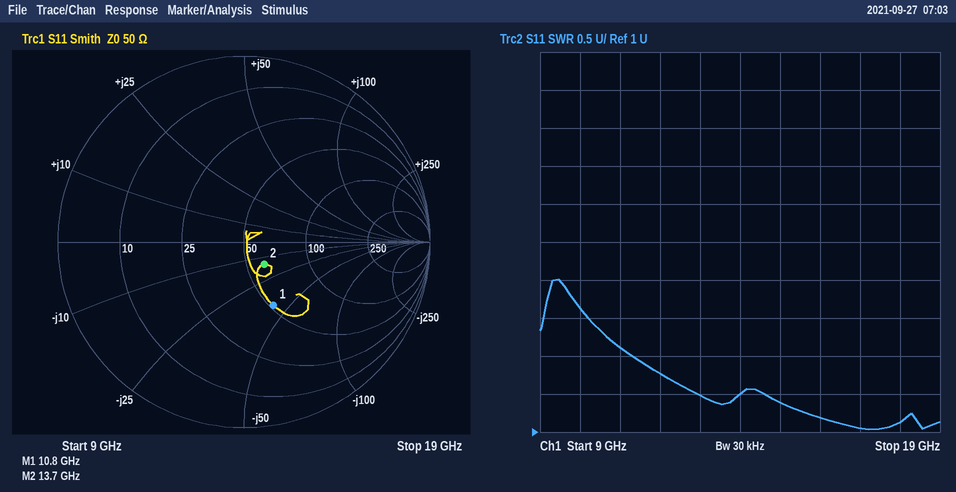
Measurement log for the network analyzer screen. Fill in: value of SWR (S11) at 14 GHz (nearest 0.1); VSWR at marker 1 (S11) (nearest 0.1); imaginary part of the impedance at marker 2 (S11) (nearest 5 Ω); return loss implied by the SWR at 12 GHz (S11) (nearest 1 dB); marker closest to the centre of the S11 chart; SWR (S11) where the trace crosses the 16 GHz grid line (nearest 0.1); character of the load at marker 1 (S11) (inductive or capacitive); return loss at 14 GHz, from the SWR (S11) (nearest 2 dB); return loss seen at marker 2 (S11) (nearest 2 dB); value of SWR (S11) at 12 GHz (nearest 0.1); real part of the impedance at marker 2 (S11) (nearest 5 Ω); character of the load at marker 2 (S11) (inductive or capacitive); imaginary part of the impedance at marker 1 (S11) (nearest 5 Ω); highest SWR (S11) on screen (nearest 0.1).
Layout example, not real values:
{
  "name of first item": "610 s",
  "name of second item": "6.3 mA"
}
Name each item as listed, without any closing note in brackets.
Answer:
{
  "value of SWR (S11) at 14 GHz": "1.5",
  "VSWR at marker 1 (S11)": "2.2",
  "imaginary part of the impedance at marker 2 (S11)": "-15 Ω",
  "return loss implied by the SWR at 12 GHz (S11)": "11 dB",
  "marker closest to the centre of the S11 chart": "marker 2",
  "SWR (S11) where the trace crosses the 16 GHz grid line": "1.2",
  "character of the load at marker 1 (S11)": "capacitive",
  "return loss at 14 GHz, from the SWR (S11)": "14 dB",
  "return loss seen at marker 2 (S11)": "16 dB",
  "value of SWR (S11) at 12 GHz": "1.8",
  "real part of the impedance at marker 2 (S11)": "60 Ω",
  "character of the load at marker 2 (S11)": "capacitive",
  "imaginary part of the impedance at marker 1 (S11)": "-40 Ω",
  "highest SWR (S11) on screen": "3.0"
}
